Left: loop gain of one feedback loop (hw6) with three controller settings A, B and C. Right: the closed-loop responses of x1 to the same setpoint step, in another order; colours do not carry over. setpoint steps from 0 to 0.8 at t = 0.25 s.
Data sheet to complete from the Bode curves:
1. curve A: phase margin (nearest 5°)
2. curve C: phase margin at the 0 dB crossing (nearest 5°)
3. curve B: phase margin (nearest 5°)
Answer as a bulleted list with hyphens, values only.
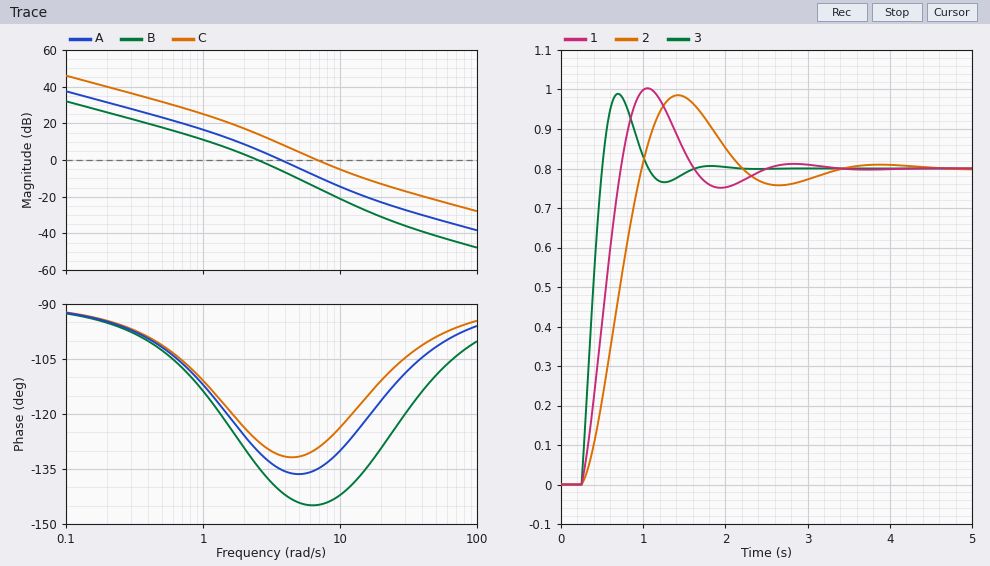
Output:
- 45°
- 50°
- 45°
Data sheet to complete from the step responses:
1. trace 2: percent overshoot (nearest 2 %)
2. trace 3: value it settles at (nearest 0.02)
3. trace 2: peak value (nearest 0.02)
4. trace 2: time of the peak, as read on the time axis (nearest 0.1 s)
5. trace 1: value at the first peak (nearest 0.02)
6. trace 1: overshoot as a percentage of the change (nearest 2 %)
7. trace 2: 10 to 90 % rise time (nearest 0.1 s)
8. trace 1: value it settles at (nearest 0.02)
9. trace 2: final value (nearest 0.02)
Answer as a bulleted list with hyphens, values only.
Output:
- 24 %
- 0.80
- 0.98
- 1.4 s
- 1.00
- 26 %
- 0.5 s
- 0.80
- 0.80
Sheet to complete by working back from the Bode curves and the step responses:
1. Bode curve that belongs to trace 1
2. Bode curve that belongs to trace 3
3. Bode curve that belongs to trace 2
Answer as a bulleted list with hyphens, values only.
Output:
- A
- C
- B
